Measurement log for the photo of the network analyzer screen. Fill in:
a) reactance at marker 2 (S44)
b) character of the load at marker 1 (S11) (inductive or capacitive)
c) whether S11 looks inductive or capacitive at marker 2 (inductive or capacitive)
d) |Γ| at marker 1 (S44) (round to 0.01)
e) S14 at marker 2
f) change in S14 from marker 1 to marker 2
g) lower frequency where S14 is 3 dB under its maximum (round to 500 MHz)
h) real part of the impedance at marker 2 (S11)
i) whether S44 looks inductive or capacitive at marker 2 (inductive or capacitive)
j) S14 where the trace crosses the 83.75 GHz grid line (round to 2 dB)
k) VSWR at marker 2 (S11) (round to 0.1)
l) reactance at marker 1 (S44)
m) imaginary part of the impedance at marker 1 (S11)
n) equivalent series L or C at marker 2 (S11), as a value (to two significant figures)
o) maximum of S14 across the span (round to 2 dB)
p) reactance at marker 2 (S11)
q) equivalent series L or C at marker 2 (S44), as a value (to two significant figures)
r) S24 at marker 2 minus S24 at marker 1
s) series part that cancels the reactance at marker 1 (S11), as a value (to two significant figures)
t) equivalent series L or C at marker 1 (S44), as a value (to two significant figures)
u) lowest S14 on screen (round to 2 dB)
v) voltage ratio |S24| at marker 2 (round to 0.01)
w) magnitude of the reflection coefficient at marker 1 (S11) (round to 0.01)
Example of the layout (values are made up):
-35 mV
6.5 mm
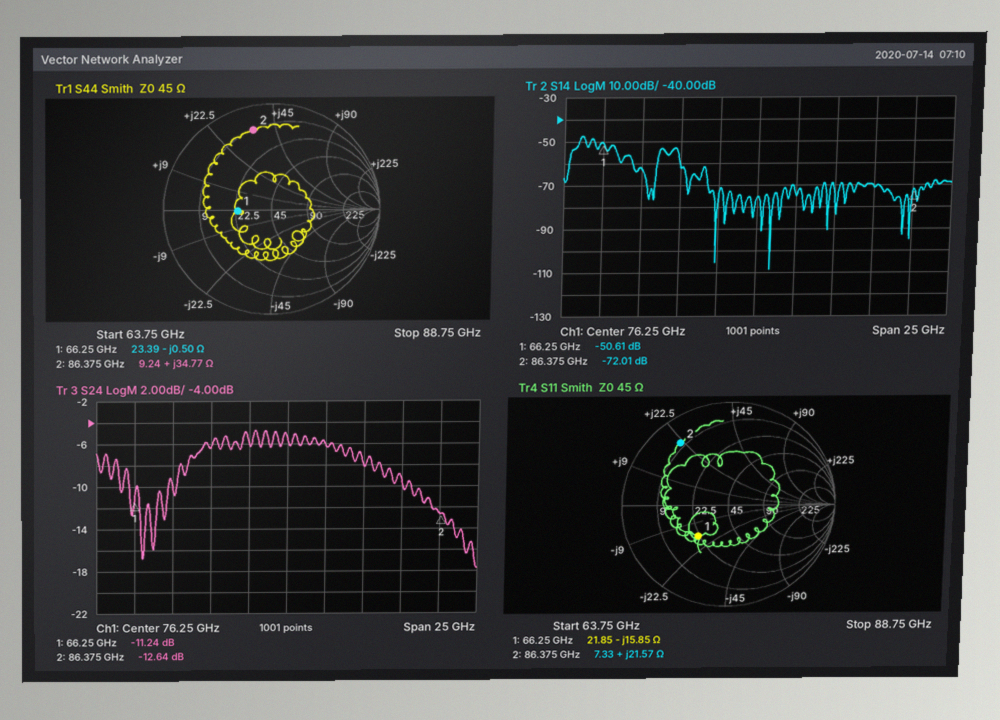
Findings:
+34.77 Ω
capacitive
inductive
0.32
-72.01 dB
-21.40 dB
64.5 GHz
7.33 Ω
inductive
-70 dB
7.6
-0.50 Ω
-15.85 Ω
40 pH
-48 dB
+21.57 Ω
64 pH
-1.40 dB
38 pH
4.8 pF
-108 dB
0.23
0.41
